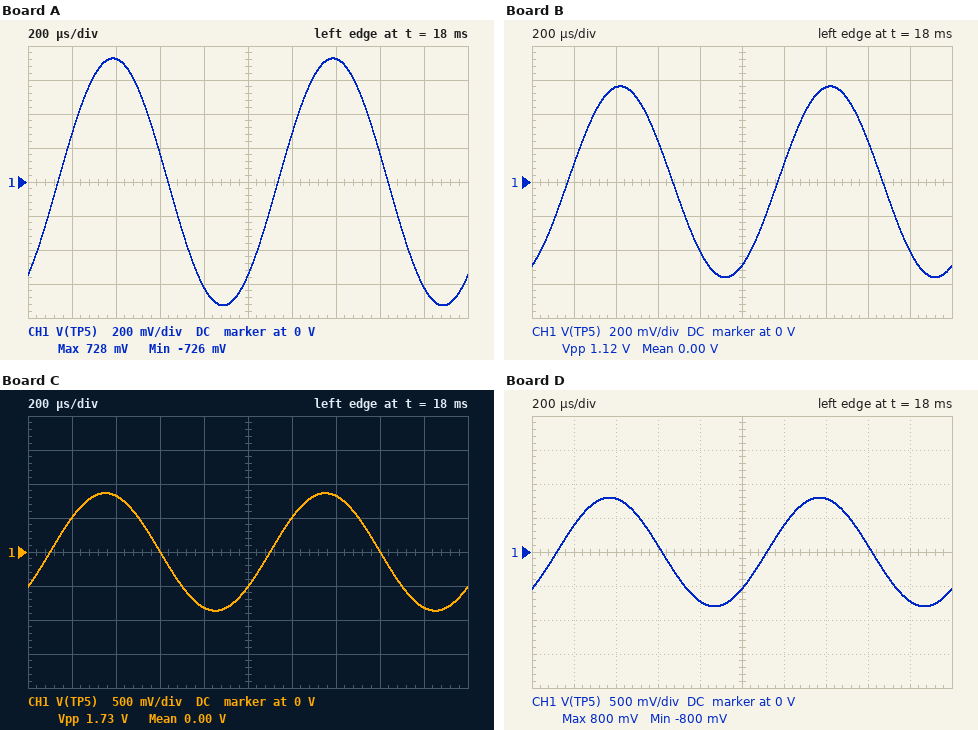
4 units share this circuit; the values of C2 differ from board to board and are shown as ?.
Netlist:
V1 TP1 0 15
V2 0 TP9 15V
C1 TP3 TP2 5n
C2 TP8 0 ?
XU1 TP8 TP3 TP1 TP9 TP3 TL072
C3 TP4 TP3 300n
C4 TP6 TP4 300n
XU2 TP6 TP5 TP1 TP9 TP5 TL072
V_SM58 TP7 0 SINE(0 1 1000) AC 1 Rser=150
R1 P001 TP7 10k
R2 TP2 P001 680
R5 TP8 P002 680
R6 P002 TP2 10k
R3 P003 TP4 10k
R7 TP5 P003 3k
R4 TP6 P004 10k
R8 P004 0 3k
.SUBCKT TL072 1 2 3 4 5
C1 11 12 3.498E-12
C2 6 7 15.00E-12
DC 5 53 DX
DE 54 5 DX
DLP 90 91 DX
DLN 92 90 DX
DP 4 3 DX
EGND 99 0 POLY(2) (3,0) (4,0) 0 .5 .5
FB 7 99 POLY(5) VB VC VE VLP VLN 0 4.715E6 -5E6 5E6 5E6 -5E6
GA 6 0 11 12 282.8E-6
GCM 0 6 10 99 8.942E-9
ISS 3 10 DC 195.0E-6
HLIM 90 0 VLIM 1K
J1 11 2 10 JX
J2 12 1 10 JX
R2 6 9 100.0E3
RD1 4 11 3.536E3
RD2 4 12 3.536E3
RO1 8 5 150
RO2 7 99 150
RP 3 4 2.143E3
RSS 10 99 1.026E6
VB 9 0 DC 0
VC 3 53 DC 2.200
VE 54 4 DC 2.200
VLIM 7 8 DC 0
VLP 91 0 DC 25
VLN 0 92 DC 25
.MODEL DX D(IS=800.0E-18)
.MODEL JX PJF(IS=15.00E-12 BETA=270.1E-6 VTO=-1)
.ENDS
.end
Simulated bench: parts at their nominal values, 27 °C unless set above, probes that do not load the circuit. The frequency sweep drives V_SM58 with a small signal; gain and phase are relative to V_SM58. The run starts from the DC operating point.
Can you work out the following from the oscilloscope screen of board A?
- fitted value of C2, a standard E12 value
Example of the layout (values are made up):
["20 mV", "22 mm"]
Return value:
["8.2 nF"]
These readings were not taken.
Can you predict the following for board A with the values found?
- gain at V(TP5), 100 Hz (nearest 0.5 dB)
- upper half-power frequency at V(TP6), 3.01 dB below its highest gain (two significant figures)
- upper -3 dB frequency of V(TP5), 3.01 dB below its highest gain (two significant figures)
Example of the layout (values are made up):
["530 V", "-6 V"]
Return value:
["-1.5 dB", "1.2 kHz", "1.2 kHz"]
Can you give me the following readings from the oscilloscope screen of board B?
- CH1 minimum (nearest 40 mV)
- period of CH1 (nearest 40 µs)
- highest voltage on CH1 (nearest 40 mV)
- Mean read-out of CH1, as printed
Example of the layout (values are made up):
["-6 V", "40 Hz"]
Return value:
["-560 mV", "1.00 ms", "560 mV", "0.00 V"]
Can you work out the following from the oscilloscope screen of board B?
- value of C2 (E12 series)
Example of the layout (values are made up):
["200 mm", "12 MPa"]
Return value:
["12 nF"]
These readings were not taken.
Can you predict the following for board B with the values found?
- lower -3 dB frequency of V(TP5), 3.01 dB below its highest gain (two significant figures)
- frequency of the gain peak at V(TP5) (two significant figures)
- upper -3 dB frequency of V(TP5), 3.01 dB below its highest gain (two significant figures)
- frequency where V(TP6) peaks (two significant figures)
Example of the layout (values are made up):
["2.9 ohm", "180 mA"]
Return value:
["56 Hz", "200 Hz", "790 Hz", "200 Hz"]
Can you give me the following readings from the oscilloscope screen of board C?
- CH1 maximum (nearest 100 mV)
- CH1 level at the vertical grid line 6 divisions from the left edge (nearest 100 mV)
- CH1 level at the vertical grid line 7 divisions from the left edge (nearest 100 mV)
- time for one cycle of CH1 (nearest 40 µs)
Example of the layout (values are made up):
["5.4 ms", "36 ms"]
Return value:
["900 mV", "500 mV", "800 mV", "1.00 ms"]
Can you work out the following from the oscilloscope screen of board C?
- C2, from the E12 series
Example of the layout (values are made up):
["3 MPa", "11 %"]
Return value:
["5.6 nF"]
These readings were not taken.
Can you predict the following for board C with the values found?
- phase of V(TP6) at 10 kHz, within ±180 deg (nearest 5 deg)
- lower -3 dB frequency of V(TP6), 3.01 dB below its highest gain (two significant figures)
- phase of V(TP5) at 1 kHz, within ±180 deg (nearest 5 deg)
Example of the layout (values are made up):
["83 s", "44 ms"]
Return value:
["-145 deg", "60 Hz", "-35 deg"]
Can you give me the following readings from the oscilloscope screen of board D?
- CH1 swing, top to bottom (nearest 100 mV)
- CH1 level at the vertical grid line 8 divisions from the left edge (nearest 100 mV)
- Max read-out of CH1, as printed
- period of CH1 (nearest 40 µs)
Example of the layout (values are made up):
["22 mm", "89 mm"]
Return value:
["1.6 V", "100 mV", "800 mV", "1.00 ms"]
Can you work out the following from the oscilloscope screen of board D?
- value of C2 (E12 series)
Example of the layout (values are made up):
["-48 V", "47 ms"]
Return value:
["6.8 nF"]
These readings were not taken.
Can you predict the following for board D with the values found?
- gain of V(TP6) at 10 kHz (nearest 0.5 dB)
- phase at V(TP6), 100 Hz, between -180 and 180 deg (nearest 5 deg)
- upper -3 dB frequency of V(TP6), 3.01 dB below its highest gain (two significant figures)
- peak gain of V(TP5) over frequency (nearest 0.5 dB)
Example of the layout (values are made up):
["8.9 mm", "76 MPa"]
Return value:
["-24.5 dB", "40 deg", "1.4 kHz", "-0.5 dB"]
